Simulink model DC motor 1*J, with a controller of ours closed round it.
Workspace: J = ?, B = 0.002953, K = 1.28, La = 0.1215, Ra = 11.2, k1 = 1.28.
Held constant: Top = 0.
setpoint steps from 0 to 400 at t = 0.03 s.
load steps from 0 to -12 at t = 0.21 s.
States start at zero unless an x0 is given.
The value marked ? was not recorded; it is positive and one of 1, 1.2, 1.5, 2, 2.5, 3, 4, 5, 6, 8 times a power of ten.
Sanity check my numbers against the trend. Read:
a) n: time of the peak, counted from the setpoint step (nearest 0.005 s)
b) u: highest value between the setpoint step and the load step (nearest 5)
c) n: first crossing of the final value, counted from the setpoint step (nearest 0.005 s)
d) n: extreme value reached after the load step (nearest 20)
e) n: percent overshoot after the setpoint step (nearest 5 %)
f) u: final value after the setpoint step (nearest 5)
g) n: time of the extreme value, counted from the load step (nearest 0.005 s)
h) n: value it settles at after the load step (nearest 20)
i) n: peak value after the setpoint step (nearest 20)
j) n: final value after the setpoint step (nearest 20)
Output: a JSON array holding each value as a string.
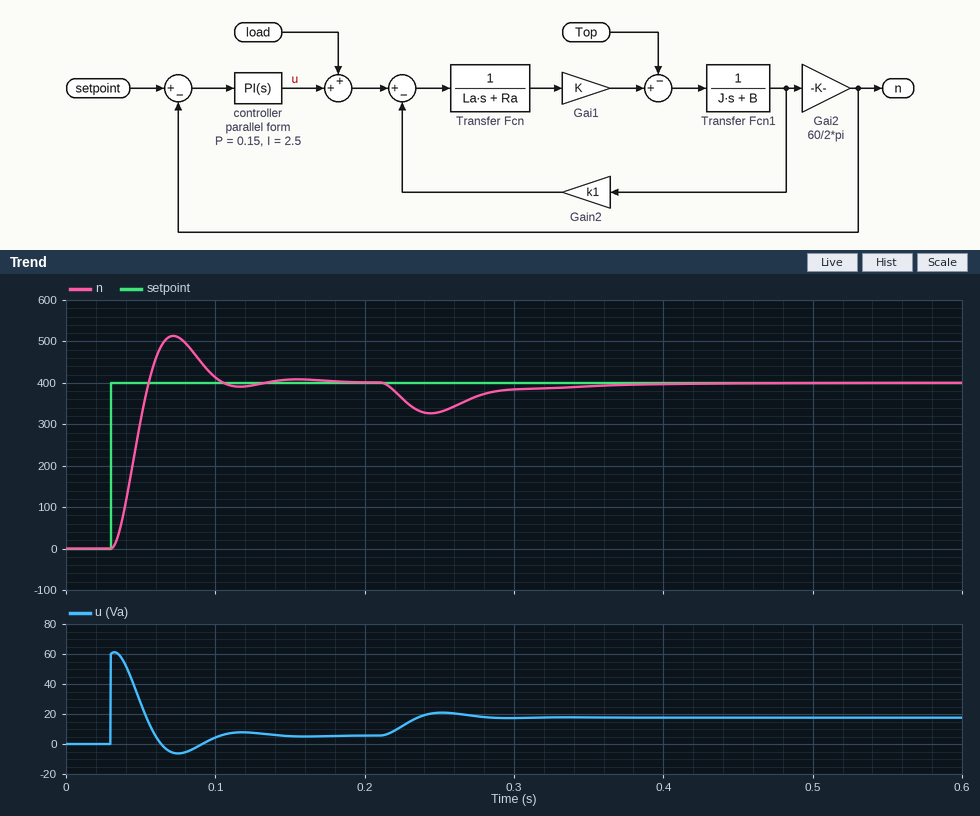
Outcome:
["0.040 s", "60", "0.025 s", "320", "30 %", "5", "0.035 s", "400", "520", "400"]
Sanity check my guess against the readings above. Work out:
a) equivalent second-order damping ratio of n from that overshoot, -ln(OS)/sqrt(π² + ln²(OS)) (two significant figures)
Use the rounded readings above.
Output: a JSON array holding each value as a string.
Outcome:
["0.36"]
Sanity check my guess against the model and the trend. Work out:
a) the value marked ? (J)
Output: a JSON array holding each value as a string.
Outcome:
["0.02"]
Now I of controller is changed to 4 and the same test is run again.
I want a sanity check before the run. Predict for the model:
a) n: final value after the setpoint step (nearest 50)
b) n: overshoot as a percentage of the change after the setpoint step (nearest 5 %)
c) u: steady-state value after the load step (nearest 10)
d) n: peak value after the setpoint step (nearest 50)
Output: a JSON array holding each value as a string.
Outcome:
["400", "40 %", "20", "550"]
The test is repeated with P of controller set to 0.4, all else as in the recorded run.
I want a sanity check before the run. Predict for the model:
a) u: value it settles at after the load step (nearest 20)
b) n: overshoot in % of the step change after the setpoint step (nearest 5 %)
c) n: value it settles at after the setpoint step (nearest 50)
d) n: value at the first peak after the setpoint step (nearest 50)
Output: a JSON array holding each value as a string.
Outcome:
["20", "35 %", "400", "550"]
